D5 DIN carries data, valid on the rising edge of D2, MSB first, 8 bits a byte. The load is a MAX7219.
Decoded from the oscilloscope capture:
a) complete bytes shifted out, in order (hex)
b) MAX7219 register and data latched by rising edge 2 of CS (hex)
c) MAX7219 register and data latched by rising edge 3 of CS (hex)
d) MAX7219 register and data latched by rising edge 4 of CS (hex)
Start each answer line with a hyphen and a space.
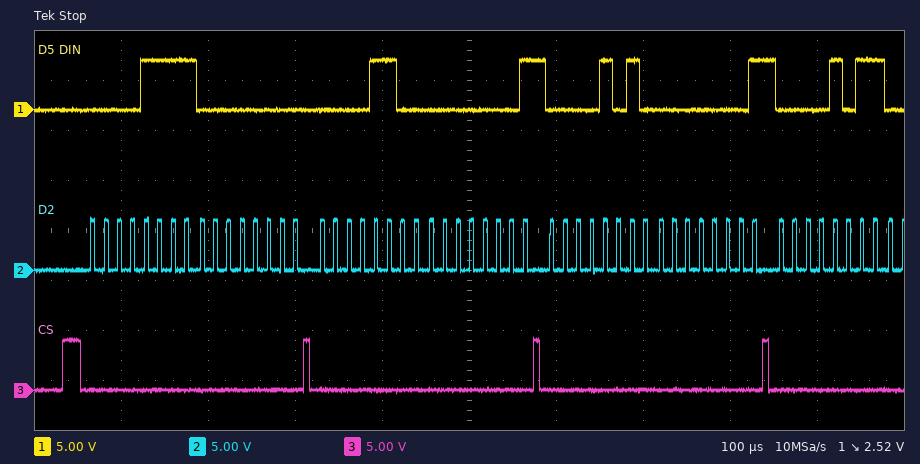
- 0F 00 0C 01 0A 01 0B
- register 0xF, data 0x00
- register 0xC, data 0x01
- register 0xA, data 0x01
